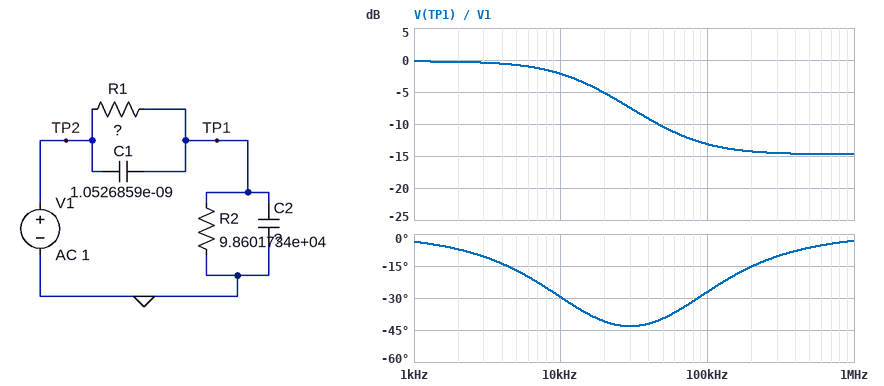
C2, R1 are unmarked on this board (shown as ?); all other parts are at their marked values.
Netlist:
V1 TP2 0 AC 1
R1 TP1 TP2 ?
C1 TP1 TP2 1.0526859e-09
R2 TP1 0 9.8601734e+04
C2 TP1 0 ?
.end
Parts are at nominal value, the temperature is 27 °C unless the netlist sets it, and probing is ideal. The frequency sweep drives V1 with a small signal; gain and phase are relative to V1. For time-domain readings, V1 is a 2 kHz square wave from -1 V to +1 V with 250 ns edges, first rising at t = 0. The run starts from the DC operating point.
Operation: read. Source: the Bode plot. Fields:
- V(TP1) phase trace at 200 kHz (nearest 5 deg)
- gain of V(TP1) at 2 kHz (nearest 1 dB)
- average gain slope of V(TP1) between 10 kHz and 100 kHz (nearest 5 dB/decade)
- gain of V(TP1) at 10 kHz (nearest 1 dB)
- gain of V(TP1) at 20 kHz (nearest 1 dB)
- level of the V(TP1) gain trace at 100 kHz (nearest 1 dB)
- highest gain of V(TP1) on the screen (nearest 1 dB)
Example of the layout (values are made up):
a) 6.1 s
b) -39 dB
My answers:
a) -15 deg
b) 0 dB
c) -10 dB/decade
d) -2 dB
e) -5 dB
f) -13 dB
g) 0 dB
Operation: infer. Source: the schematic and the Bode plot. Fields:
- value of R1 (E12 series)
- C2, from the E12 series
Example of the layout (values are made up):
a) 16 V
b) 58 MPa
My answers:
a) 2.2 kΩ
b) 4.7 nF
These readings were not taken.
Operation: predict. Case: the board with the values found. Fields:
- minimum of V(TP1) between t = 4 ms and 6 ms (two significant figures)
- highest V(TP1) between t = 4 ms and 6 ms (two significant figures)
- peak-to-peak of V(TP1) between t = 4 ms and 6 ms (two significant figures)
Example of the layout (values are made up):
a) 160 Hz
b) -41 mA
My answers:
a) -980 mV
b) 980 mV
c) 2.0 V
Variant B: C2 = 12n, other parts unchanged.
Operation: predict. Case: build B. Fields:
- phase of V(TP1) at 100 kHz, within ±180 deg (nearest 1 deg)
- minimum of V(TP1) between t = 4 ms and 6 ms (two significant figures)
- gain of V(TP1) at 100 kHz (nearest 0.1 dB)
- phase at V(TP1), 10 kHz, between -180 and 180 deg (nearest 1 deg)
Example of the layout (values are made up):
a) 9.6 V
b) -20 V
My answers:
a) -31 deg
b) -980 mV
c) -20.2 dB
d) -52 deg
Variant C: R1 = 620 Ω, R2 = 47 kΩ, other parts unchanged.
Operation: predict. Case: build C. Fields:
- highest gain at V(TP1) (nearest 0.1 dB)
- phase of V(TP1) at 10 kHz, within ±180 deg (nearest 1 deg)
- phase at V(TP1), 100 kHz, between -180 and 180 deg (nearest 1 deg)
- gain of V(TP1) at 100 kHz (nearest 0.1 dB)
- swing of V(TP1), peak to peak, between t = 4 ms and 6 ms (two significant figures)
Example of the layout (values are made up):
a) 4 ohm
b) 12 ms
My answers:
a) -0.1 dB
b) -10 deg
c) -43 deg
d) -7.1 dB
e) 2.0 V
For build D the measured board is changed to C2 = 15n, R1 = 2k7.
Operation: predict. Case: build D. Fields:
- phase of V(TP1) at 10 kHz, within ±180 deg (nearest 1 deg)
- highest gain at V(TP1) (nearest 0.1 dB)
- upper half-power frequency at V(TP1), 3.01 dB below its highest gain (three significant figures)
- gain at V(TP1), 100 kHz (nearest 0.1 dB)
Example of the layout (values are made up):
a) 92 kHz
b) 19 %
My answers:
a) -59 deg
b) -0.2 dB
c) 3.79 kHz
d) -22.5 dB
